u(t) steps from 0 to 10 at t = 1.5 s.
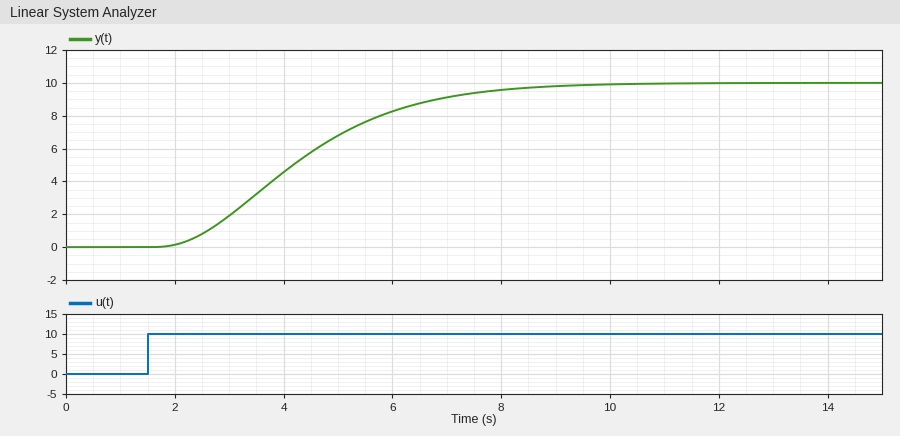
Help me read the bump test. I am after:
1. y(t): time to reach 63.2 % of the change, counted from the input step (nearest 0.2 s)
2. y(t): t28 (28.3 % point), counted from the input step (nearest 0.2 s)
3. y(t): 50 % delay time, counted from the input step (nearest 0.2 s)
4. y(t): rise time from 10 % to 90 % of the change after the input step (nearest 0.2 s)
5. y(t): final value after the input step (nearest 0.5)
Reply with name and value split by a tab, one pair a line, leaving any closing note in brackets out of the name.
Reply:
y(t): time to reach 63.2 % of the change, counted from the input step	3.2 s
y(t): t28 (28.3 % point), counted from the input step	1.8 s
y(t): 50 % delay time, counted from the input step	2.6 s
y(t): rise time from 10 % to 90 % of the change after the input step	4.2 s
y(t): final value after the input step	10.0
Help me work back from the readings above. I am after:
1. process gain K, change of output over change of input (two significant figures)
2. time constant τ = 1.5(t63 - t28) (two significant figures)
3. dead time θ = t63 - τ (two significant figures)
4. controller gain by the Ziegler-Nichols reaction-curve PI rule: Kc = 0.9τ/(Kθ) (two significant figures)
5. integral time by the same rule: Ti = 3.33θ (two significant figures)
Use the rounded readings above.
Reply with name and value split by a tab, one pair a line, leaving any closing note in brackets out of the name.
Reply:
process gain K, change of output over change of input	1.0
time constant τ = 1.5(t63 - t28)	2.1 s
dead time θ = t63 - τ	1.1 s
controller gain by the Ziegler-Nichols reaction-curve PI rule: Kc = 0.9τ/(Kθ)	1.7
integral time by the same rule: Ti = 3.33θ	3.7 s
